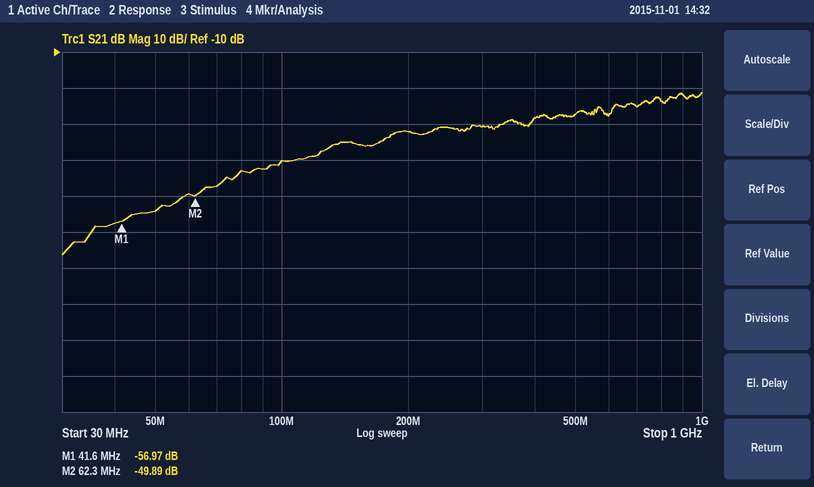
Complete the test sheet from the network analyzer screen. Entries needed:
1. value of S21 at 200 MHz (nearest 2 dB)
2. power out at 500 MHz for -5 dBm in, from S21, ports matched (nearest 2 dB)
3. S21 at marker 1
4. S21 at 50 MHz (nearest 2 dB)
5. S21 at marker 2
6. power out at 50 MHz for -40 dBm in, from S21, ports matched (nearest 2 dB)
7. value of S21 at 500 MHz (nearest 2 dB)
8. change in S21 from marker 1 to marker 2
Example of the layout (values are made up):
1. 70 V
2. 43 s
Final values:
1. -32 dB
2. -32 dBm
3. -56.97 dB
4. -54 dB
5. -49.89 dB
6. -94 dBm
7. -28 dB
8. 7.08 dB
